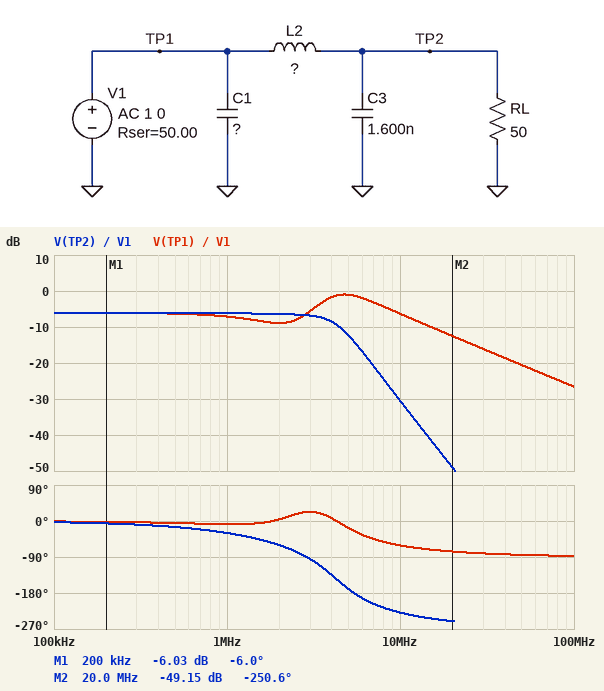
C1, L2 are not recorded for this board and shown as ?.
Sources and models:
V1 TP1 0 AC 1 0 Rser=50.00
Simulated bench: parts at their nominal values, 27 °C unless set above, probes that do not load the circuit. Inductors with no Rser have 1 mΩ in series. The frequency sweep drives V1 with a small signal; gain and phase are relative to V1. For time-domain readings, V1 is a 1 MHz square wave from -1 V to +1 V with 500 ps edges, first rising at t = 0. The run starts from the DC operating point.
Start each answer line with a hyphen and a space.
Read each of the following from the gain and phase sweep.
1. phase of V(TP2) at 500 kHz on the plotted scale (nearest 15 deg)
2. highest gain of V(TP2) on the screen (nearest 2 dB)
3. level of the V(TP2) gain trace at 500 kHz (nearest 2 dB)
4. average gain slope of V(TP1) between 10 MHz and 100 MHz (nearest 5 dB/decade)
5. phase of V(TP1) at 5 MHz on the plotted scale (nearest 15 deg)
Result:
- -15 deg
- -6 dB
- -6 dB
- -20 dB/decade
- -15 deg
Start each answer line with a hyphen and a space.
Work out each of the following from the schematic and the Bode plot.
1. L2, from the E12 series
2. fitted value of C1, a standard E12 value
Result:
- 2.7 µH
- 680 pF
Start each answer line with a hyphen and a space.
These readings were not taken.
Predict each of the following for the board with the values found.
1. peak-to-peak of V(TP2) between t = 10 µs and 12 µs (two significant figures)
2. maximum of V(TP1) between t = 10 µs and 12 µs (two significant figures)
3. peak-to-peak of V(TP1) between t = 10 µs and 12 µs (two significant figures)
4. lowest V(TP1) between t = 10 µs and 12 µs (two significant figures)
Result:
- 1.1 V
- 730 mV
- 1.5 V
- -730 mV
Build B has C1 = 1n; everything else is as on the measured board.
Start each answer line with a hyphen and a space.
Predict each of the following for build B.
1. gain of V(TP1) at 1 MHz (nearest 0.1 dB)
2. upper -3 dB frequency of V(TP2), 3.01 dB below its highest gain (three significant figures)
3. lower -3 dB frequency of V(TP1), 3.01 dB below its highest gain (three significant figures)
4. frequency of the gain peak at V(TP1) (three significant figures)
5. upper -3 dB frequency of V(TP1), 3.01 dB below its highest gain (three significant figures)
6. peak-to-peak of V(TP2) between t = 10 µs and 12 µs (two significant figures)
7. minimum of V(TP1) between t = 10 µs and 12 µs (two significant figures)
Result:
- -7.2 dB
- 4.08 MHz
- 3.07 MHz
- 4.16 MHz
- 6.20 MHz
- 1.2 V
- -630 mV
